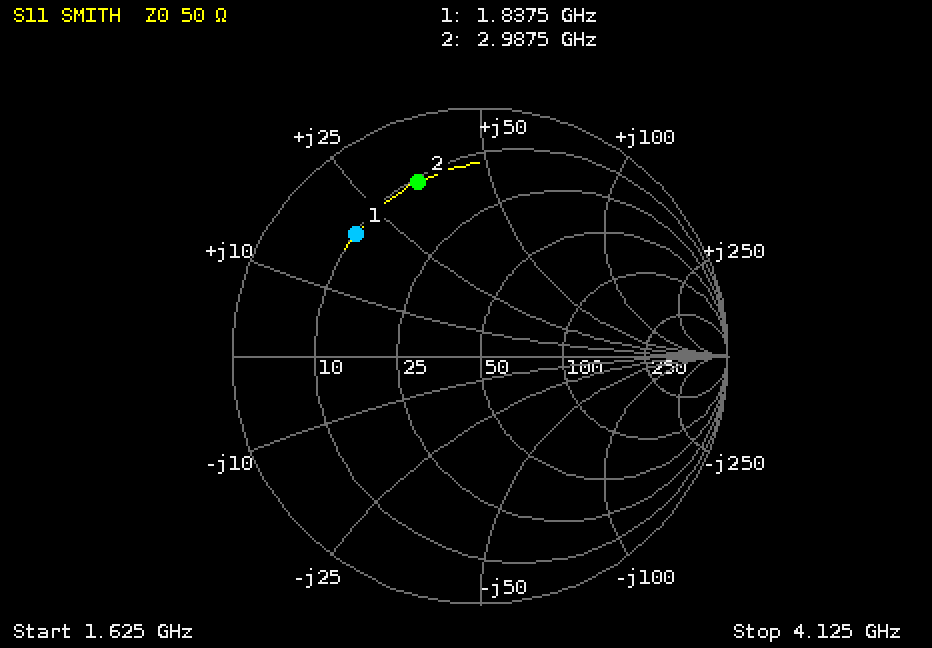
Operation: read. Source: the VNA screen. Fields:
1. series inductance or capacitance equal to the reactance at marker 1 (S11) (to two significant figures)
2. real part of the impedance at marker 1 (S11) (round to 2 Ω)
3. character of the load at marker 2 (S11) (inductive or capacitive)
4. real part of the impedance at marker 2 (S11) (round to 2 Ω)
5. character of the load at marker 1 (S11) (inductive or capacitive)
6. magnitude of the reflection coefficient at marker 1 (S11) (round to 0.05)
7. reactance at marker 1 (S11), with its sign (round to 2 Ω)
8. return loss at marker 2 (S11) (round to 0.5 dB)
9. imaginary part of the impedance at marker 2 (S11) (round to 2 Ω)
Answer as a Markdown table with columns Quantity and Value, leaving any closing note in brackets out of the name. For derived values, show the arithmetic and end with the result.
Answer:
| Quantity | Value |
|---|---|
| series inductance or capacitance equal to the reactance at marker 1 (S11) | L = 20 Ω/(2π × 1.8375 GHz) ≈ 1.7 nH |
| real part of the impedance at marker 1 (S11) | 10 Ω |
| character of the load at marker 2 (S11) | inductive |
| real part of the impedance at marker 2 (S11) | 10 Ω |
| character of the load at marker 1 (S11) | inductive |
| magnitude of the reflection coefficient at marker 1 (S11) | 0.70 |
| reactance at marker 1 (S11), with its sign | +20 Ω |
| return loss at marker 2 (S11) | 2.5 dB |
| imaginary part of the impedance at marker 2 (S11) | +34 Ω |
